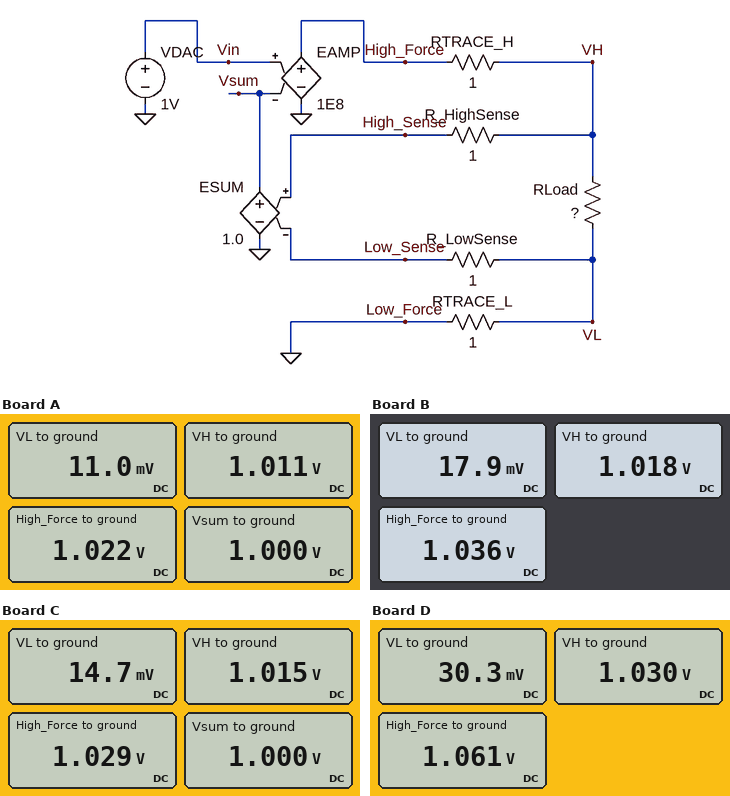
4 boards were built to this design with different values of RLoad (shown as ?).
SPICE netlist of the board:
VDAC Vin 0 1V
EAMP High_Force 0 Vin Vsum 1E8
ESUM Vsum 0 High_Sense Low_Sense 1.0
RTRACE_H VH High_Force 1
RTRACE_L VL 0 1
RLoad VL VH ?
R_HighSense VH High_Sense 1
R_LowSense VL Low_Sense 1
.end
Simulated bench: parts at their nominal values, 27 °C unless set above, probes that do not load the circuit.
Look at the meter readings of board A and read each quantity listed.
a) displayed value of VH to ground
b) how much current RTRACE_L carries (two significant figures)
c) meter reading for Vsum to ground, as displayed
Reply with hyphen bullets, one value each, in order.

- 1.011 V
- 11 mA
- 1.000 V
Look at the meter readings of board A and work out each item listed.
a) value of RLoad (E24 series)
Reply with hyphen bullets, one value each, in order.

- 91 Ω
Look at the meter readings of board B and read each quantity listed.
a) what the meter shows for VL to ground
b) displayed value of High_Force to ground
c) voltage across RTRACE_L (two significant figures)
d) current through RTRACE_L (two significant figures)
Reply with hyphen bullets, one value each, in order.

- 17.9 mV
- 1.036 V
- 18 mV
- 18 mA
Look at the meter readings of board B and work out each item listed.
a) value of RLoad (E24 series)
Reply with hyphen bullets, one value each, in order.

- 56 Ω
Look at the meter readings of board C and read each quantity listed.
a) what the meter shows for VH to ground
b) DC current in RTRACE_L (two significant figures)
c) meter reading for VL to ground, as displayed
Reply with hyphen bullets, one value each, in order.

- 1.015 V
- 15 mA
- 14.7 mV
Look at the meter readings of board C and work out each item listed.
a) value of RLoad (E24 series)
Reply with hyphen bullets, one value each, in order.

- 68 Ω
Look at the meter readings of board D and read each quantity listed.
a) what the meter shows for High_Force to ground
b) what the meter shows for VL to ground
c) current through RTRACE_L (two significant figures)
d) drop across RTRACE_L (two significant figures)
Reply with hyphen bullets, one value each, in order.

- 1.061 V
- 30.3 mV
- 30 mA
- 30 mV
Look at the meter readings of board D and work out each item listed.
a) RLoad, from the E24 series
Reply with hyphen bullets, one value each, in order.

- 33 Ω
